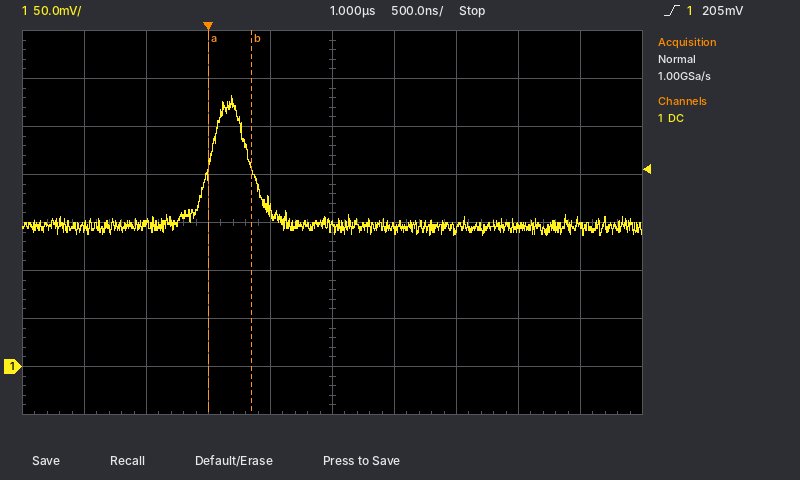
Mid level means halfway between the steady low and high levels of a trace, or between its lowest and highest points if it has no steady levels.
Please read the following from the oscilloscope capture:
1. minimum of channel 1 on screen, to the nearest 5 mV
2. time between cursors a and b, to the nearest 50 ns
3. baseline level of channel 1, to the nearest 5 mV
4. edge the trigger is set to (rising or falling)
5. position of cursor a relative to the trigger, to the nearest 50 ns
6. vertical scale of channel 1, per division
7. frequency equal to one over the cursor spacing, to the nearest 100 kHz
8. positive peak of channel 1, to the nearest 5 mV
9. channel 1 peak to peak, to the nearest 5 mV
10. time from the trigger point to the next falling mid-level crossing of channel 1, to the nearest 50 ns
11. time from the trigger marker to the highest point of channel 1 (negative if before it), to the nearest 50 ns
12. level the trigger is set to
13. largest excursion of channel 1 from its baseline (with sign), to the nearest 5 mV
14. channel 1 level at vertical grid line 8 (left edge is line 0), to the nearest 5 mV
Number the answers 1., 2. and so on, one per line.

1. 135 mV
2. 350 ns
3. 145 mV
4. rising
5. 0 ns
6. 50 mV
7. 2.9 MHz
8. 280 mV
9. 145 mV
10. 350 ns
11. +200 ns
12. 205 mV
13. +135 mV
14. 145 mV
